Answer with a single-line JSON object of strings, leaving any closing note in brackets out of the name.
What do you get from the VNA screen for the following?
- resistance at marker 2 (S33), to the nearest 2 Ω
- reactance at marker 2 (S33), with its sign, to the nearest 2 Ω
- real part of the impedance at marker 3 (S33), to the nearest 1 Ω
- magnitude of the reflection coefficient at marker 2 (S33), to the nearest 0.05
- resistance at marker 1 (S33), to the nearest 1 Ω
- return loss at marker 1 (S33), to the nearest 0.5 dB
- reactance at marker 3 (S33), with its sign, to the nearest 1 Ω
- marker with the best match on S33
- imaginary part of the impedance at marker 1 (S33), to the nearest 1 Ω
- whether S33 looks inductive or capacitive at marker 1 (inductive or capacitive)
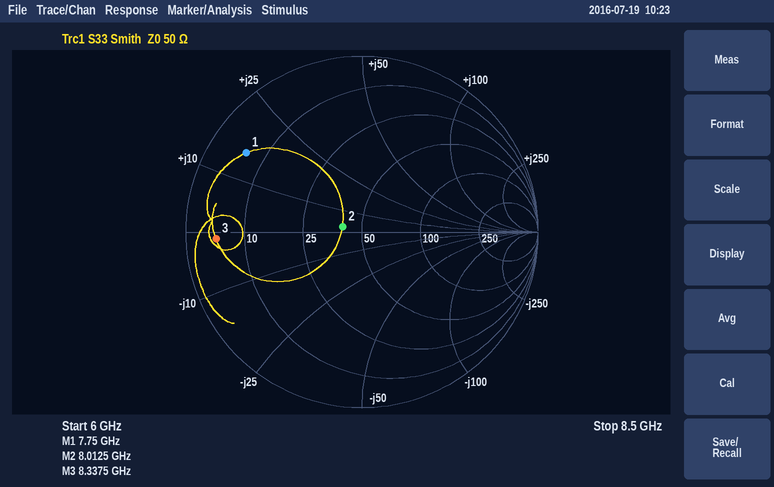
{"resistance at marker 2 (S33), to the nearest 2 Ω": "40 Ω", "reactance at marker 2 (S33), with its sign, to the nearest 2 Ω": "+2 Ω", "real part of the impedance at marker 3 (S33), to the nearest 1 Ω": "5 Ω", "magnitude of the reflection coefficient at marker 2 (S33), to the nearest 0.05": "0.10", "resistance at marker 1 (S33), to the nearest 1 Ω": "6 Ω", "return loss at marker 1 (S33), to the nearest 0.5 dB": "2.0 dB", "reactance at marker 3 (S33), with its sign, to the nearest 1 Ω": "-1 Ω", "marker with the best match on S33": "marker 2", "imaginary part of the impedance at marker 1 (S33), to the nearest 1 Ω": "+15 Ω", "whether S33 looks inductive or capacitive at marker 1": "inductive"}
